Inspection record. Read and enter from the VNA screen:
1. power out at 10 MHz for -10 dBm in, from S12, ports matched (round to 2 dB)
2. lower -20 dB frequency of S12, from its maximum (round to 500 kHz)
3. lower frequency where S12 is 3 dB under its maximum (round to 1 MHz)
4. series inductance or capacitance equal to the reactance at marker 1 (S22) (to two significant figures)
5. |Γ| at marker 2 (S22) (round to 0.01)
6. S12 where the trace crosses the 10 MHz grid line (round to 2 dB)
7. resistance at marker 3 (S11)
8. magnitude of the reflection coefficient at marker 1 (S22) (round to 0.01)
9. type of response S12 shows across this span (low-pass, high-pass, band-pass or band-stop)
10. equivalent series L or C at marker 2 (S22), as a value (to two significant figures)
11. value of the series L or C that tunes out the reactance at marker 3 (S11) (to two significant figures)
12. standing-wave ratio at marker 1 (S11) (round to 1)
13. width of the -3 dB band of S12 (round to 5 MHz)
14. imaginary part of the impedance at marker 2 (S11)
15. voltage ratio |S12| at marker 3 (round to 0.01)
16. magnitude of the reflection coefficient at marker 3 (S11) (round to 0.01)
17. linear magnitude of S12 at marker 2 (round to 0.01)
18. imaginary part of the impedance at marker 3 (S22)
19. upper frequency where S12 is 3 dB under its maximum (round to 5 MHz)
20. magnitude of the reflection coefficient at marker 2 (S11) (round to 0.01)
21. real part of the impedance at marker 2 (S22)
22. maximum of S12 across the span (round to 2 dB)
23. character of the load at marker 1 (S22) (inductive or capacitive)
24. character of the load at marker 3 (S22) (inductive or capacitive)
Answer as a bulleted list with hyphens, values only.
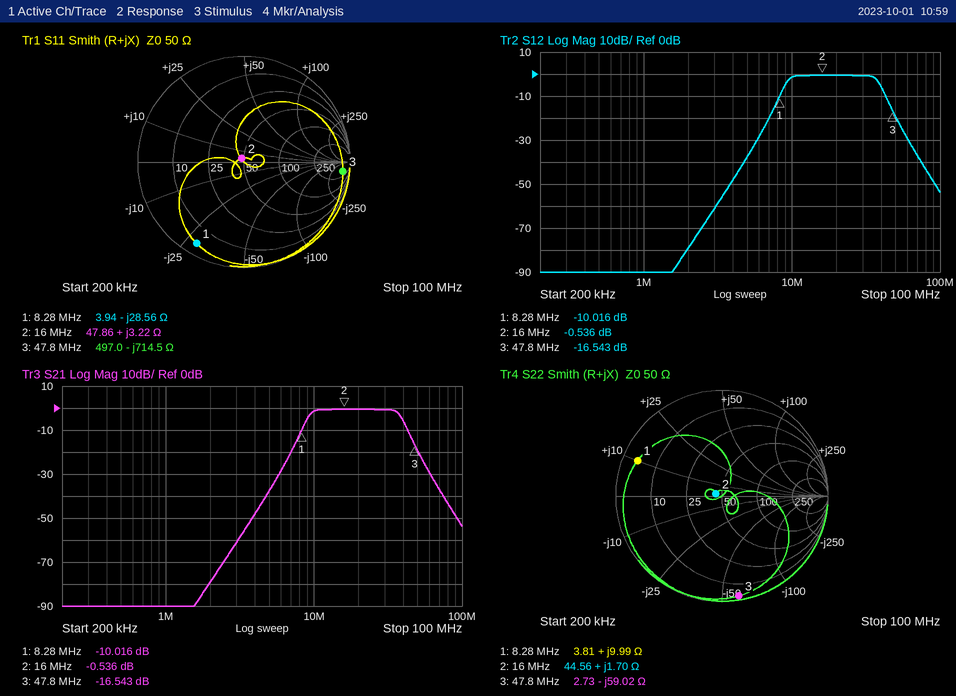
- -12 dBm
- 7.0 MHz
- 9 MHz
- 190 nH
- 0.06
- -2 dB
- 497.0 Ω
- 0.86
- band-pass
- 17 nH
- 2.4 µH
- 17
- 30 MHz
- +3.22 Ω
- 0.15
- 0.94
- 0.94
- -59.02 Ω
- 40 MHz
- 0.04
- 44.56 Ω
- 0 dB
- inductive
- capacitive
